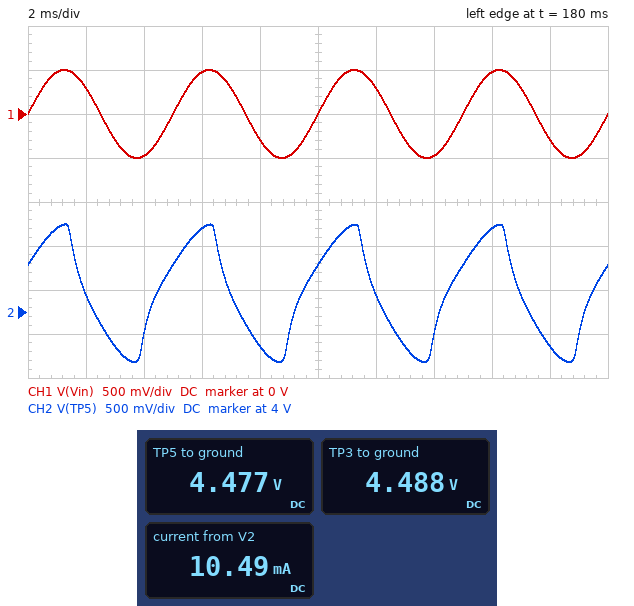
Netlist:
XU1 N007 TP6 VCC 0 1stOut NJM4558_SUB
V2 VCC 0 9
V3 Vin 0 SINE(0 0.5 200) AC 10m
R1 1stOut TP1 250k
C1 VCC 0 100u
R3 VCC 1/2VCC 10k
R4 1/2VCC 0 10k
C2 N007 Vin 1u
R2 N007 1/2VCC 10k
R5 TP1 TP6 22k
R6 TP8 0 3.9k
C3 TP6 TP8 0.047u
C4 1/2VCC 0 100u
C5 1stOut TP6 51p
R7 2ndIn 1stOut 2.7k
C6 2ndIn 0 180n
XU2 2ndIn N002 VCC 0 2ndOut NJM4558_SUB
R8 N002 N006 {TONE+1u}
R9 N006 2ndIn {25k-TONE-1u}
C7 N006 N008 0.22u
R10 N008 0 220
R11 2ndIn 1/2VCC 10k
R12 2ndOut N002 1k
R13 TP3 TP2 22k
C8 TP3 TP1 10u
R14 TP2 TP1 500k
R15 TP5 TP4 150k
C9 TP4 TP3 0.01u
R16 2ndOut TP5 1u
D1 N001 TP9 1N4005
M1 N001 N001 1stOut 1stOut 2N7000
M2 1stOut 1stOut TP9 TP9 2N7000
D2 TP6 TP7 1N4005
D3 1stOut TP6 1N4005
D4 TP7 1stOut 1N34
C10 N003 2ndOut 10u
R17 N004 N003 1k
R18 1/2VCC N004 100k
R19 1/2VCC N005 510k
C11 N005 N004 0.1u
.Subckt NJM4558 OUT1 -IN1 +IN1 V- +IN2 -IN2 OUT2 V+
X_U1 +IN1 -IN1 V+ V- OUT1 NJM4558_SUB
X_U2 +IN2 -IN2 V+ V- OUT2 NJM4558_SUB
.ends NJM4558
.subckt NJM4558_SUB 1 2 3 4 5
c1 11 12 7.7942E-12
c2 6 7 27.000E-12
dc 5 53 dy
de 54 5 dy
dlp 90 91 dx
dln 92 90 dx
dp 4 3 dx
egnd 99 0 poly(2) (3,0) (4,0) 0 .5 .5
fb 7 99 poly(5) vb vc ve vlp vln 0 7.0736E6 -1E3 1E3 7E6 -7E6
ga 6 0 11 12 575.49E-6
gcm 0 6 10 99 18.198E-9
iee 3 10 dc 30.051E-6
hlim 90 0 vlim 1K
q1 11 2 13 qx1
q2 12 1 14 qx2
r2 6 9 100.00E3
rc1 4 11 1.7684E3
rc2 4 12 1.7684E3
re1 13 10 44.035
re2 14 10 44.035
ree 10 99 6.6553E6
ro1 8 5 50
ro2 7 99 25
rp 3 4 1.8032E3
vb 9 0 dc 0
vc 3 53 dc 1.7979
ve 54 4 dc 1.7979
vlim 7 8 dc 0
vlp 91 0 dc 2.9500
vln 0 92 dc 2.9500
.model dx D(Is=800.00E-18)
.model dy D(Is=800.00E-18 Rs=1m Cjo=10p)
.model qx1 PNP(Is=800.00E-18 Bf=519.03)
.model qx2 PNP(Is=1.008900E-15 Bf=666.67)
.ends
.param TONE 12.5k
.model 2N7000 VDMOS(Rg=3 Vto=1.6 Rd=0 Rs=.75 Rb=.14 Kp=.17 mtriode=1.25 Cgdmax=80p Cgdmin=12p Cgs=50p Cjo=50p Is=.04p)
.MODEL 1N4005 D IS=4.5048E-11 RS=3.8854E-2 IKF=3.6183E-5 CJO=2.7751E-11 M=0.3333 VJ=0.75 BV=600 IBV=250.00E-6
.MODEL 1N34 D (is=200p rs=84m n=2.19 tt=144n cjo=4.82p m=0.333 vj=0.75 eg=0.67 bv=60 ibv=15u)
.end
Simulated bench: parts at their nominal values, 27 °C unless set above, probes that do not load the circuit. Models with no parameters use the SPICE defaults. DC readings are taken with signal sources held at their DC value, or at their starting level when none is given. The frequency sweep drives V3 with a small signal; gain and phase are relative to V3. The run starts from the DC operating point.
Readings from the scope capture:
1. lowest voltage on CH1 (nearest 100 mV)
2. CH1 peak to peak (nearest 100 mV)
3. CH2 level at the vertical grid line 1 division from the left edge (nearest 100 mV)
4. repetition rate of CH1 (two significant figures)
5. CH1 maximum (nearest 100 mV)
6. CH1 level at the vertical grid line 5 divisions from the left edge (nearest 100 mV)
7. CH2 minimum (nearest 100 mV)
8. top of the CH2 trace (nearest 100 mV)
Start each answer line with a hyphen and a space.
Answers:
- -500 mV
- 1.0 V
- 4.2 V
- 200 Hz
- 500 mV
- 0 V
- 3.4 V
- 5.0 V
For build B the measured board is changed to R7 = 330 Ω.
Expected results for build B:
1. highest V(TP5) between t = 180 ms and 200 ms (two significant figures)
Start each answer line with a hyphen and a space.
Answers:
- 5.3 V
